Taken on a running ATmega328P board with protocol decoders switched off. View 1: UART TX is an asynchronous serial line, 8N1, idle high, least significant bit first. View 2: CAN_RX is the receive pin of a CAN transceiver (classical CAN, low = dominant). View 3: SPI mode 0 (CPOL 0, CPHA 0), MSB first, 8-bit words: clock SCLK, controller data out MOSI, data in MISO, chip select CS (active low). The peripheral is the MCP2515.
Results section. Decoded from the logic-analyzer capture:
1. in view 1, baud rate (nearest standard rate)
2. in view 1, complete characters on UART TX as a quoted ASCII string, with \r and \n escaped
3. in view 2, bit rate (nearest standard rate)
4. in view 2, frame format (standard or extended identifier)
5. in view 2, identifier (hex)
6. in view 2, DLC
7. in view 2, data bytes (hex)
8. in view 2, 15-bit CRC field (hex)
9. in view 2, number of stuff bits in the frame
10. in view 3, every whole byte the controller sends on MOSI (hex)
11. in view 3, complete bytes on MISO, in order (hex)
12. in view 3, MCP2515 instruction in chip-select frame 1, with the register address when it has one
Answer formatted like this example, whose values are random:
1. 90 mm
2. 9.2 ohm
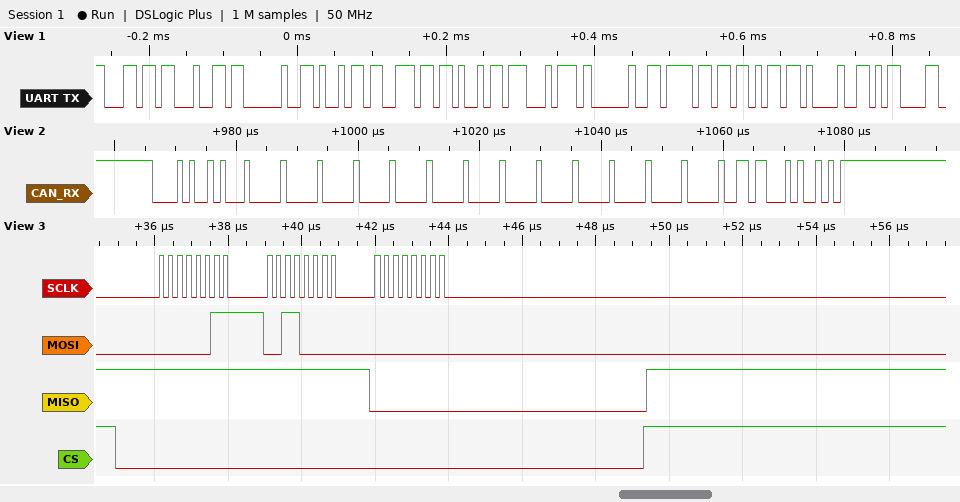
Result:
1. 115200 baud
2. "ld init ok!\r"
3. 1000 kbit/s
4. standard
5. 0x0A5
6. 8
7. 00 00 00 00 00 00 00 00
8. 0x6C52
9. 13
10. 0x03 0x30 0x00
11. 0xFF 0xFF 0x00
12. READ 0x30
